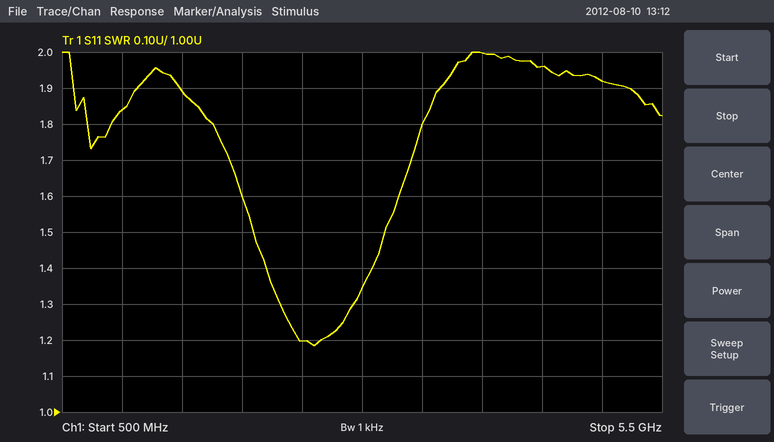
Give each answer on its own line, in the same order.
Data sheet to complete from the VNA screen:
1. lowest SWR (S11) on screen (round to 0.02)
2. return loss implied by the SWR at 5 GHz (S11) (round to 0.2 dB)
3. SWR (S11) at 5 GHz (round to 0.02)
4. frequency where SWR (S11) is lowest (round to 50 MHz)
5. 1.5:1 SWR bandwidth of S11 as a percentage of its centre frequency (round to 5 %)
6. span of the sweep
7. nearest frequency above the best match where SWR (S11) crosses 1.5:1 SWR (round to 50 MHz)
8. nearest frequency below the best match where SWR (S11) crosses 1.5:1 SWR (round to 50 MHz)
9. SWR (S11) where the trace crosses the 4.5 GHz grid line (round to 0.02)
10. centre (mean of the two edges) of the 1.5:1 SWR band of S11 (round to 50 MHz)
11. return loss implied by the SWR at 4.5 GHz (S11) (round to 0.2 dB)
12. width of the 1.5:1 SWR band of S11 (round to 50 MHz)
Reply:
1.18
10.0 dB
1.92
2.60 GHz
40 %
5 GHz
3.20 GHz
2.10 GHz
1.96
2.65 GHz
9.8 dB
1.10 GHz
